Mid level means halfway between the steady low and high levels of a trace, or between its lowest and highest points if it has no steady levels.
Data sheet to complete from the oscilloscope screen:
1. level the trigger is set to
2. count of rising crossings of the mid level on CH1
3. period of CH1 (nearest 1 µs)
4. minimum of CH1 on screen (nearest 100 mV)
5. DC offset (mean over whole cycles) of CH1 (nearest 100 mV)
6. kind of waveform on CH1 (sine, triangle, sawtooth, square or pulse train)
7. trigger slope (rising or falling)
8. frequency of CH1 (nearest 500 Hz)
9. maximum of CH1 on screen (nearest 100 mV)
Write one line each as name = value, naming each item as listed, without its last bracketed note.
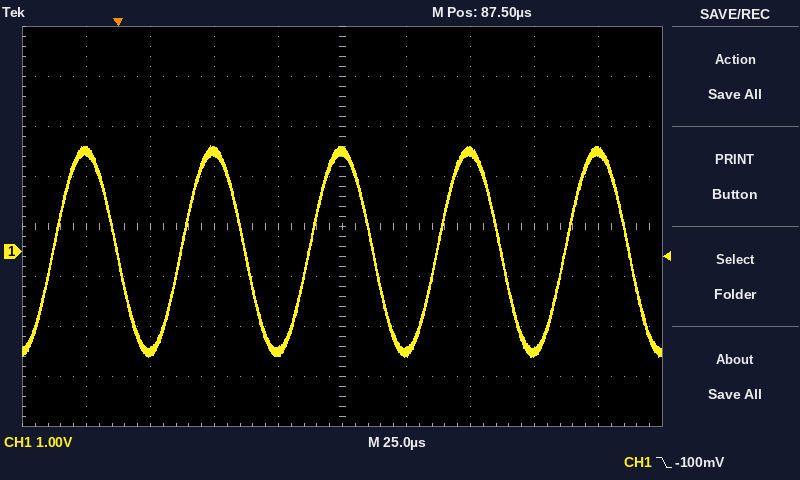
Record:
level the trigger is set to = -100 mV
count of rising crossings of the mid level on CH1 = 5
period of CH1 = 50 µs
minimum of CH1 on screen = -2.1 V
DC offset (mean over whole cycles) of CH1 = 0.0 V
kind of waveform on CH1 = sine
trigger slope = falling
frequency of CH1 = 20.0 kHz
maximum of CH1 on screen = 2.1 V
